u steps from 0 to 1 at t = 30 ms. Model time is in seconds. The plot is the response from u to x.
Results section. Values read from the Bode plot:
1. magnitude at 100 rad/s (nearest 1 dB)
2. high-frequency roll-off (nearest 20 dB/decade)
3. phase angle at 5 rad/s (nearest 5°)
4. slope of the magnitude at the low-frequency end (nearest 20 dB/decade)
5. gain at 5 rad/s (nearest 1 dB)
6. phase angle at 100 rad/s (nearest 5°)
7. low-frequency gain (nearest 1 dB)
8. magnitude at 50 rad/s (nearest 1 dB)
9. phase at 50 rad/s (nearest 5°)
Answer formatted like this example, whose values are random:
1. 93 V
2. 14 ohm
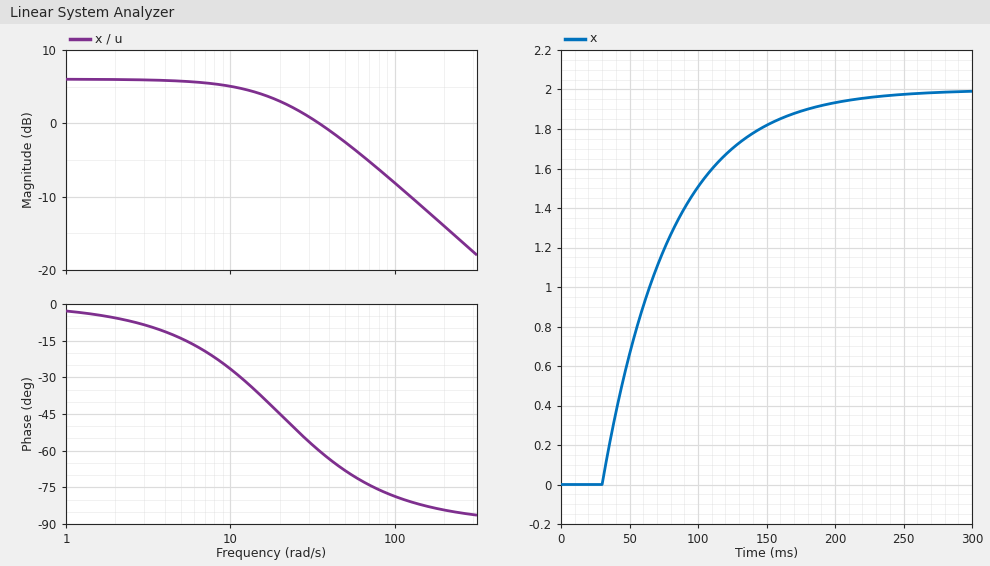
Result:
1. -8 dB
2. -20 dB/decade
3. -15°
4. 0 dB/decade
5. 6 dB
6. -80°
7. 6 dB
8. -3 dB
9. -70°
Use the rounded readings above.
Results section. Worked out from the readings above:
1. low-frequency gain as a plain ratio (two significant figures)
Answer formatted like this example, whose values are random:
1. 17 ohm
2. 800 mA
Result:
1. 2.0
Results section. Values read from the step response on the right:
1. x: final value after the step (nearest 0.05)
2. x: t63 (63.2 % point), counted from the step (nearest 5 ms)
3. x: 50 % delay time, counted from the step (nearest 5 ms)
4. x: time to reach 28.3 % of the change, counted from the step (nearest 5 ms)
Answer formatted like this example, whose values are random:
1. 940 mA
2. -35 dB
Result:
1. 2.00
2. 50 ms
3. 35 ms
4. 15 ms
